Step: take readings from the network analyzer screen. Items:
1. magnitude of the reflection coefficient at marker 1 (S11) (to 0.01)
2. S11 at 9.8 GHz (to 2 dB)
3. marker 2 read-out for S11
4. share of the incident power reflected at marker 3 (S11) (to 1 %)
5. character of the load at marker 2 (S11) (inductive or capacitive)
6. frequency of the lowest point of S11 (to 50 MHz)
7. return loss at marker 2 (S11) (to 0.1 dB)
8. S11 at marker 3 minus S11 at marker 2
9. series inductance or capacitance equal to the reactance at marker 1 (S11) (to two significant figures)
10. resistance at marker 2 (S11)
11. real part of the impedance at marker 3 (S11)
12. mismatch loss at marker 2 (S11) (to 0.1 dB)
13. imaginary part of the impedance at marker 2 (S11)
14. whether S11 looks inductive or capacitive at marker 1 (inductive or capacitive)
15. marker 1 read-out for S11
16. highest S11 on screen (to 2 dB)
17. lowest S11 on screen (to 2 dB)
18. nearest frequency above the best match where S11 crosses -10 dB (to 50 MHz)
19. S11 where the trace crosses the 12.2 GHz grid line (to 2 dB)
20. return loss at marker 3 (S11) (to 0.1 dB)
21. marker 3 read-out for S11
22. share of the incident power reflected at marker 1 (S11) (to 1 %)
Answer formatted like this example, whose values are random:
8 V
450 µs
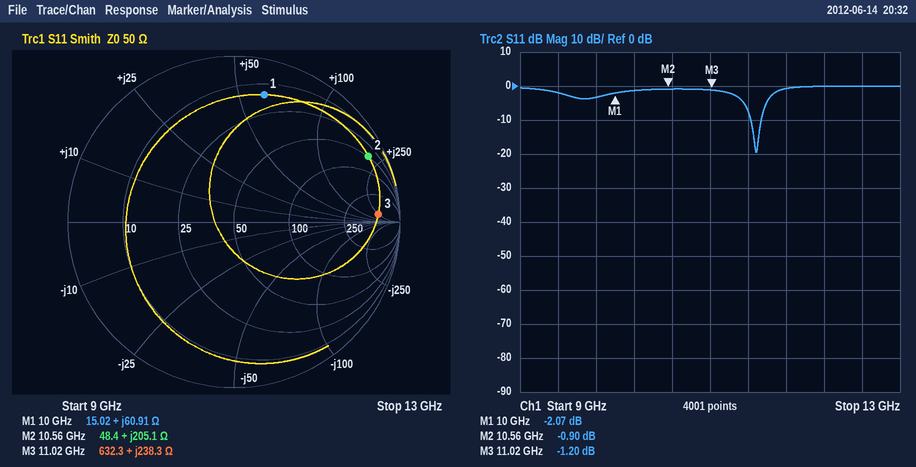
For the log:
0.79
-4 dB
-0.90 dB
76 %
inductive
11.50 GHz
0.9 dB
-0.30 dB
970 pH
48.4 Ω
632.3 Ω
7.3 dB
+205.1 Ω
inductive
-2.07 dB
0 dB
-20 dB
11.55 GHz
0 dB
1.2 dB
-1.20 dB
62 %
